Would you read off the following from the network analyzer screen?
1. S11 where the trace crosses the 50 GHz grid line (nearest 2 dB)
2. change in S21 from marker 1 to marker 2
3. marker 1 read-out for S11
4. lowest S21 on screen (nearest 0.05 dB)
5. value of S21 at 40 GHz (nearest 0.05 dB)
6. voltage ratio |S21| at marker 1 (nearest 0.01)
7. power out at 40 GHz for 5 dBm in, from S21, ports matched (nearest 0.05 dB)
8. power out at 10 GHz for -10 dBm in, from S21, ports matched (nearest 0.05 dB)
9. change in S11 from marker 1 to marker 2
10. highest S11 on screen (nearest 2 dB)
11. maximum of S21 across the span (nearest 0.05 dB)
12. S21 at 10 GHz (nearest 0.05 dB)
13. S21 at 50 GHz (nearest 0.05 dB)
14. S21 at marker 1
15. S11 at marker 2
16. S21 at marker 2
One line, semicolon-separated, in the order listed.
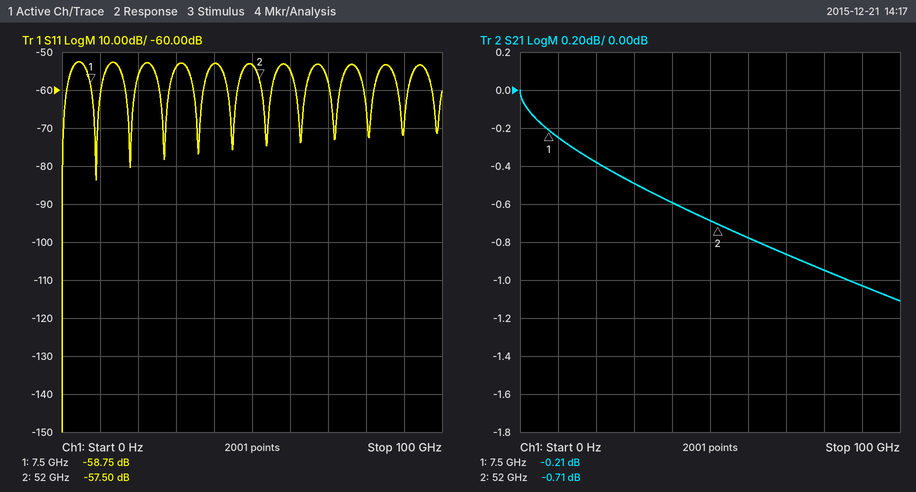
-54 dB; -0.50 dB; -58.75 dB; -1.10 dB; -0.60 dB; 0.98; 4.40 dBm; -10.25 dBm; 1.25 dB; -52 dB; 0.00 dB; -0.25 dB; -0.70 dB; -0.21 dB; -57.50 dB; -0.71 dB
